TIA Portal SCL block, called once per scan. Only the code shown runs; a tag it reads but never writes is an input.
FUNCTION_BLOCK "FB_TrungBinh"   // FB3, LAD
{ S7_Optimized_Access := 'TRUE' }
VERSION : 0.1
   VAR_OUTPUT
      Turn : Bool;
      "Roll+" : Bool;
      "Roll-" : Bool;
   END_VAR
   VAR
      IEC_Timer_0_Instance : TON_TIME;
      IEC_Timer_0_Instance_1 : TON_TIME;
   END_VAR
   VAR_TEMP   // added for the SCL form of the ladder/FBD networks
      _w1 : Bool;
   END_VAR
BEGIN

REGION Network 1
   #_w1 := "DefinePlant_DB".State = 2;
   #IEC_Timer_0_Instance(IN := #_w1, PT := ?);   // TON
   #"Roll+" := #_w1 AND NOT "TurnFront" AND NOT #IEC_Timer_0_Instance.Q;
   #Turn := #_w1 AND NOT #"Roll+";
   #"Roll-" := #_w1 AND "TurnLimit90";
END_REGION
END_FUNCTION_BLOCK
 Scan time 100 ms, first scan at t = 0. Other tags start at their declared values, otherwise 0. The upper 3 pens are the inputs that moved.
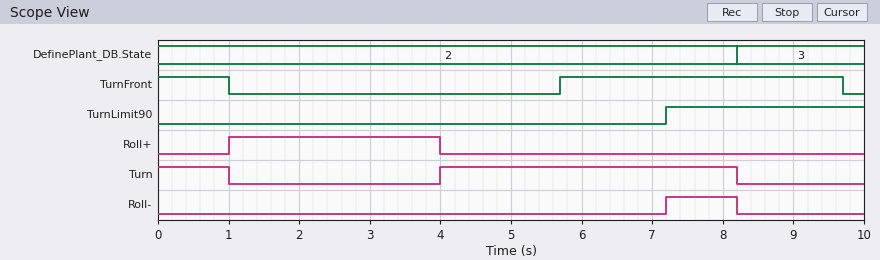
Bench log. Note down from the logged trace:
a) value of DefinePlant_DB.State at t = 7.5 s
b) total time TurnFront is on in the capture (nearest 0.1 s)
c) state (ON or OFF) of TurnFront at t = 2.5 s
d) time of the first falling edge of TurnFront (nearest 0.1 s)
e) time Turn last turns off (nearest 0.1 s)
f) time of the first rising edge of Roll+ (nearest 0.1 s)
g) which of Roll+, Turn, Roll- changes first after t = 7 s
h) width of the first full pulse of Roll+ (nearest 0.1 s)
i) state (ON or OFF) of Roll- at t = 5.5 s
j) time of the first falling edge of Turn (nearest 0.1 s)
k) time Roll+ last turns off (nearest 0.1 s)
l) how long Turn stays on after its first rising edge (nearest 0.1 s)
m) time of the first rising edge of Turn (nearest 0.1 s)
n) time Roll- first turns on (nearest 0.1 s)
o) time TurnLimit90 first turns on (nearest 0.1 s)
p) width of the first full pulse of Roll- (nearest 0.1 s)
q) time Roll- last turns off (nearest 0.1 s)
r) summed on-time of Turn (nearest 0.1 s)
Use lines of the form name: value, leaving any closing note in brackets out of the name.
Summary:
value of DefinePlant_DB.State at t = 7.5 s: 2
total time TurnFront is on in the capture: 5.0 s
state (ON or OFF) of TurnFront at t = 2.5 s: OFF
time of the first falling edge of TurnFront: 1.0 s
time Turn last turns off: 8.2 s
time of the first rising edge of Roll+: 1.0 s
which of Roll+, Turn, Roll- changes first after t = 7 s: Roll-
width of the first full pulse of Roll+: 3.0 s
state (ON or OFF) of Roll- at t = 5.5 s: OFF
time of the first falling edge of Turn: 1.0 s
time Roll+ last turns off: 4.0 s
how long Turn stays on after its first rising edge: 4.2 s
time of the first rising edge of Turn: 4.0 s
time Roll- first turns on: 7.2 s
time TurnLimit90 first turns on: 7.2 s
width of the first full pulse of Roll-: 1.0 s
time Roll- last turns off: 8.2 s
summed on-time of Turn: 5.2 s
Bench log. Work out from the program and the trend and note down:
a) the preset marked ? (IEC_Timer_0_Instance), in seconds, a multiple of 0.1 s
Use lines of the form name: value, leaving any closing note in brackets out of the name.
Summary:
the preset marked ? (IEC_Timer_0_Instance), in seconds, a multiple of 0.1 s: 4.0 s
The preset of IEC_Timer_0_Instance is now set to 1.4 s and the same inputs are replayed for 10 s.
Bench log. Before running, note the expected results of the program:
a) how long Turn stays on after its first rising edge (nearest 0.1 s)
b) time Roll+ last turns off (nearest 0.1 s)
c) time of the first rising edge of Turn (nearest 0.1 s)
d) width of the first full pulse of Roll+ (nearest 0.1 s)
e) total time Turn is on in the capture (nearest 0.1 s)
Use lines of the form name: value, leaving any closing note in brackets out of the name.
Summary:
how long Turn stays on after its first rising edge: 6.8 s
time Roll+ last turns off: 1.4 s
time of the first rising edge of Turn: 1.4 s
width of the first full pulse of Roll+: 0.4 s
total time Turn is on in the capture: 7.8 s
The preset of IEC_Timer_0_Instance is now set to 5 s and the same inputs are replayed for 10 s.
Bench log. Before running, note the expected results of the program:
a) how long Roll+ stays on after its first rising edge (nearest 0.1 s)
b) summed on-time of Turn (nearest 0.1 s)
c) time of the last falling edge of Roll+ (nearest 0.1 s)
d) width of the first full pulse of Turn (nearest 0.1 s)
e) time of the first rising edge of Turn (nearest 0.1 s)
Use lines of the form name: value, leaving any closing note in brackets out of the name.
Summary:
how long Roll+ stays on after its first rising edge: 4.0 s
summed on-time of Turn: 4.2 s
time of the last falling edge of Roll+: 5.0 s
width of the first full pulse of Turn: 3.2 s
time of the first rising edge of Turn: 5.0 s
